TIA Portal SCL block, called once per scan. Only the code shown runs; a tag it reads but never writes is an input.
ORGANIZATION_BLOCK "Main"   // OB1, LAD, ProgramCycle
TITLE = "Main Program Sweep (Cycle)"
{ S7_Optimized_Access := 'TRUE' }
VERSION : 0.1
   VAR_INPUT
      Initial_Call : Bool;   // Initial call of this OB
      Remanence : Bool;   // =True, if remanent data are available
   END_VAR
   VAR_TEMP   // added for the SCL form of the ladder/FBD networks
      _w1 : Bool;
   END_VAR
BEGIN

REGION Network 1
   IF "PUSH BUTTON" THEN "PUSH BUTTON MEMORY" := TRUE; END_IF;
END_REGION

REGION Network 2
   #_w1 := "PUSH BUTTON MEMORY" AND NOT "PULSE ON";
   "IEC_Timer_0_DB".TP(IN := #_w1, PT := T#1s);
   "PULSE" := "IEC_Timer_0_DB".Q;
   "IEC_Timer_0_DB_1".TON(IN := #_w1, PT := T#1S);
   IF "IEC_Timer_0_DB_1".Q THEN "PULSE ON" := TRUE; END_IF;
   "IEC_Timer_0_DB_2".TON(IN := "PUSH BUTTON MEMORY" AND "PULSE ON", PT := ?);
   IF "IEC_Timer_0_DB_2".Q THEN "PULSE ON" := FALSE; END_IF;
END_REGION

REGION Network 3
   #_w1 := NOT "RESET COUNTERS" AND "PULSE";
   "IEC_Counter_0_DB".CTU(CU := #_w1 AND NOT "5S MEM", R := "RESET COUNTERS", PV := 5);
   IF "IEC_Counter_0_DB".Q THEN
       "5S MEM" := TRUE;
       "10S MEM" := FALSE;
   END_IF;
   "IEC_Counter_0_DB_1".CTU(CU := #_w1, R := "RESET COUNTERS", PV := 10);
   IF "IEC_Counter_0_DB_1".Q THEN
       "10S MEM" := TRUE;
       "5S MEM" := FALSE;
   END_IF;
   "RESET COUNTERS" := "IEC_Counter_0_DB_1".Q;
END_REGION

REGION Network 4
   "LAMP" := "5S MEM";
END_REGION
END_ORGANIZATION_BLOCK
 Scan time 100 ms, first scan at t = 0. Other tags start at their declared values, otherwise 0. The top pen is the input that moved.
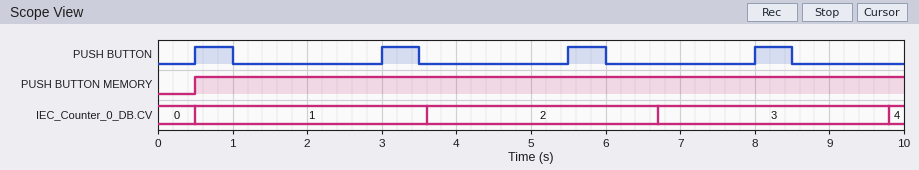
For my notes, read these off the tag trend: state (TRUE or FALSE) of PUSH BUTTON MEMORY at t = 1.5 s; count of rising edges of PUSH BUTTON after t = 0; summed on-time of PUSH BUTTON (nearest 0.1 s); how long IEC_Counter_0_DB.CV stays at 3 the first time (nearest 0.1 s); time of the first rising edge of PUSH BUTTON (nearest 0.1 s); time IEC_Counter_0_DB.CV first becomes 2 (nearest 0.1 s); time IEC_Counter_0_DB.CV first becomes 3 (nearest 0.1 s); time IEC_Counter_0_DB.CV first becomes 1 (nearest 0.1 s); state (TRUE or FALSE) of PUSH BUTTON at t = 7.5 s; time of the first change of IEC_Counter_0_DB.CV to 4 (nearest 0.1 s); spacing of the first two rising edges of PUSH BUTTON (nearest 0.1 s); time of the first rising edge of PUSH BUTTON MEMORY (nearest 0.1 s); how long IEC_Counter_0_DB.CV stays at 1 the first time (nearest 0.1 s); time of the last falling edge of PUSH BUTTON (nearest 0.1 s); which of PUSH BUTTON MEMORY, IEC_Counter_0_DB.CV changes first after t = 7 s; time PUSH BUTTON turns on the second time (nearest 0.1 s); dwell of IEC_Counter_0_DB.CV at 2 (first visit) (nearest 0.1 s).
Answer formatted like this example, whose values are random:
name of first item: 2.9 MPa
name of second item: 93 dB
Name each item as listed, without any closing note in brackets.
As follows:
state (TRUE or FALSE) of PUSH BUTTON MEMORY at t = 1.5 s: TRUE
count of rising edges of PUSH BUTTON after t = 0: 4
summed on-time of PUSH BUTTON: 2.0 s
how long IEC_Counter_0_DB.CV stays at 3 the first time: 3.1 s
time of the first rising edge of PUSH BUTTON: 0.5 s
time IEC_Counter_0_DB.CV first becomes 2: 3.6 s
time IEC_Counter_0_DB.CV first becomes 3: 6.7 s
time IEC_Counter_0_DB.CV first becomes 1: 0.5 s
state (TRUE or FALSE) of PUSH BUTTON at t = 7.5 s: FALSE
time of the first change of IEC_Counter_0_DB.CV to 4: 9.8 s
spacing of the first two rising edges of PUSH BUTTON: 2.5 s
time of the first rising edge of PUSH BUTTON MEMORY: 0.5 s
how long IEC_Counter_0_DB.CV stays at 1 the first time: 3.1 s
time of the last falling edge of PUSH BUTTON: 8.5 s
which of PUSH BUTTON MEMORY, IEC_Counter_0_DB.CV changes first after t = 7 s: IEC_Counter_0_DB.CV
time PUSH BUTTON turns on the second time: 3.0 s
dwell of IEC_Counter_0_DB.CV at 2 (first visit): 3.1 s
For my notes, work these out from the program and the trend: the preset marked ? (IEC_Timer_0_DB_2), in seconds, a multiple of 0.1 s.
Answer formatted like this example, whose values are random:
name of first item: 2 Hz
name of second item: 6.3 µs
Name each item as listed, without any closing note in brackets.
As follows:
the preset marked ? (IEC_Timer_0_DB_2), in seconds, a multiple of 0.1 s: 2.0 s
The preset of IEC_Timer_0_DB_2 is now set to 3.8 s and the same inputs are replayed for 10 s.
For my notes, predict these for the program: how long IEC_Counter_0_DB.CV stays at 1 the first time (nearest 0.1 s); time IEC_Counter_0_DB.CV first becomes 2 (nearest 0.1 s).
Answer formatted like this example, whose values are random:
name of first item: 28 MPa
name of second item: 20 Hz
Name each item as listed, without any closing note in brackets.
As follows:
how long IEC_Counter_0_DB.CV stays at 1 the first time: 4.9 s
time IEC_Counter_0_DB.CV first becomes 2: 5.4 s
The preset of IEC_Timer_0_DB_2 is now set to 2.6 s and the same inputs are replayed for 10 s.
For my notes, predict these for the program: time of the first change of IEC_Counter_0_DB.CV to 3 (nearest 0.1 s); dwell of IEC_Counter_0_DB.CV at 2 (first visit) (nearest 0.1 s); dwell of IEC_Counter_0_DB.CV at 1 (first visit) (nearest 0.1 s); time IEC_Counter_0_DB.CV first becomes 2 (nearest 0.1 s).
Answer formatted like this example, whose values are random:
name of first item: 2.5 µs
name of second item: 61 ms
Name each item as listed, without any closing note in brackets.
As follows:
time of the first change of IEC_Counter_0_DB.CV to 3: 7.9 s
dwell of IEC_Counter_0_DB.CV at 2 (first visit): 3.7 s
dwell of IEC_Counter_0_DB.CV at 1 (first visit): 3.7 s
time IEC_Counter_0_DB.CV first becomes 2: 4.2 s
